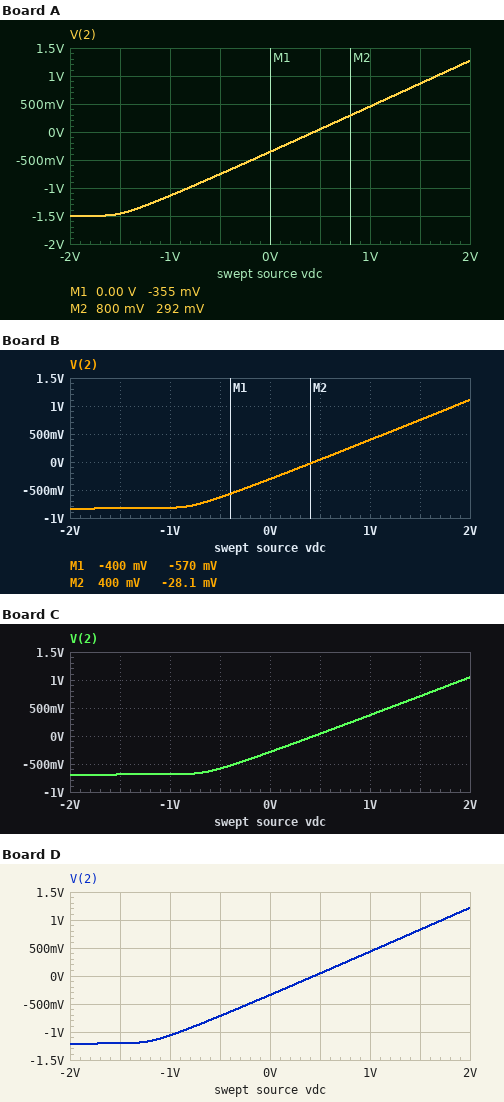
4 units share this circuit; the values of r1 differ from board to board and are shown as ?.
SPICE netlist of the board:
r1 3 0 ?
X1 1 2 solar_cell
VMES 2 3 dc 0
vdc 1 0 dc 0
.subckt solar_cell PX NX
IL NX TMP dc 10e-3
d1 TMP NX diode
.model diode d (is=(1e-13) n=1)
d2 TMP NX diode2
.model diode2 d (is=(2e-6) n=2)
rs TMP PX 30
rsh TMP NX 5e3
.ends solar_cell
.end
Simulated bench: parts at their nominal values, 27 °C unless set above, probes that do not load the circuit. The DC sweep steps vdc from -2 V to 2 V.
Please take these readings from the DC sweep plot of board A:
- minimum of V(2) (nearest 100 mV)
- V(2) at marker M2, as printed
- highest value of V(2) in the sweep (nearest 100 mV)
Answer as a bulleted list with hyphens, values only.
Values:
- -1.5 V
- 292 mV
- 1.3 V
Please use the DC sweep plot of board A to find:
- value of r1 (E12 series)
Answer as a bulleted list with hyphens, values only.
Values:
- 150 Ω
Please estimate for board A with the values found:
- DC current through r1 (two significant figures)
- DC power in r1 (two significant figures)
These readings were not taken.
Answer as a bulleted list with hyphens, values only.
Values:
- 2.4 mA
- 840 µW
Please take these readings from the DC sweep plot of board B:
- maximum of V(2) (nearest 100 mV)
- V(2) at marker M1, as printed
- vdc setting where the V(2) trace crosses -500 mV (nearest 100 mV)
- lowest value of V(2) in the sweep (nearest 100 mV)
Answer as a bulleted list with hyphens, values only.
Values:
- 1.1 V
- -570 mV
- -300 mV
- -800 mV
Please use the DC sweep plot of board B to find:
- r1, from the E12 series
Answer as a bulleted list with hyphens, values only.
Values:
- 82 Ω
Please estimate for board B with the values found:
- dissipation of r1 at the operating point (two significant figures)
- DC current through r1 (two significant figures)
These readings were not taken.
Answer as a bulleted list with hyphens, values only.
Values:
- 1.1 mW
- 3.7 mA
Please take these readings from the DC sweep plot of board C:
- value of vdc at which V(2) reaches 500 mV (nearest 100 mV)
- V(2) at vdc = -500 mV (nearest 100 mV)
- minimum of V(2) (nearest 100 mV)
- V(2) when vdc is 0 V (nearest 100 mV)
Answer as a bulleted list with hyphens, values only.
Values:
- 1.2 V
- -600 mV
- -700 mV
- -300 mV
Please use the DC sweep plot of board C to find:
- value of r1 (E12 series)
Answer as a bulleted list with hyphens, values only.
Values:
- 68 Ω
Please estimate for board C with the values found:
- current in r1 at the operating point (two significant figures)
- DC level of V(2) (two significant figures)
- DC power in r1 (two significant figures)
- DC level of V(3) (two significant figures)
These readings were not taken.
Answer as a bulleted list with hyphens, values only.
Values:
- 4.2 mA
- -290 mV
- 1.2 mW
- -290 mV
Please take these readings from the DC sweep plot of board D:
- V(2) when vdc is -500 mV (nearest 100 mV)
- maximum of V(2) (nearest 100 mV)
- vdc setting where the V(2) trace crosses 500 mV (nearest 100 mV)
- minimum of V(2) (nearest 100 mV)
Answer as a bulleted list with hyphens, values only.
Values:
- -700 mV
- 1.2 V
- 1.1 V
- -1.2 V
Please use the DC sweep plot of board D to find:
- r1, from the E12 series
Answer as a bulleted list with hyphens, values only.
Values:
- 120 Ω
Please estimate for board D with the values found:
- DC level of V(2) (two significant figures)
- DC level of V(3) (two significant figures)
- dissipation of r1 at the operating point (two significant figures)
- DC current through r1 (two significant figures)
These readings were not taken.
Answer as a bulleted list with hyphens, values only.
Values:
- -340 mV
- -340 mV
- 950 µW
- 2.8 mA
